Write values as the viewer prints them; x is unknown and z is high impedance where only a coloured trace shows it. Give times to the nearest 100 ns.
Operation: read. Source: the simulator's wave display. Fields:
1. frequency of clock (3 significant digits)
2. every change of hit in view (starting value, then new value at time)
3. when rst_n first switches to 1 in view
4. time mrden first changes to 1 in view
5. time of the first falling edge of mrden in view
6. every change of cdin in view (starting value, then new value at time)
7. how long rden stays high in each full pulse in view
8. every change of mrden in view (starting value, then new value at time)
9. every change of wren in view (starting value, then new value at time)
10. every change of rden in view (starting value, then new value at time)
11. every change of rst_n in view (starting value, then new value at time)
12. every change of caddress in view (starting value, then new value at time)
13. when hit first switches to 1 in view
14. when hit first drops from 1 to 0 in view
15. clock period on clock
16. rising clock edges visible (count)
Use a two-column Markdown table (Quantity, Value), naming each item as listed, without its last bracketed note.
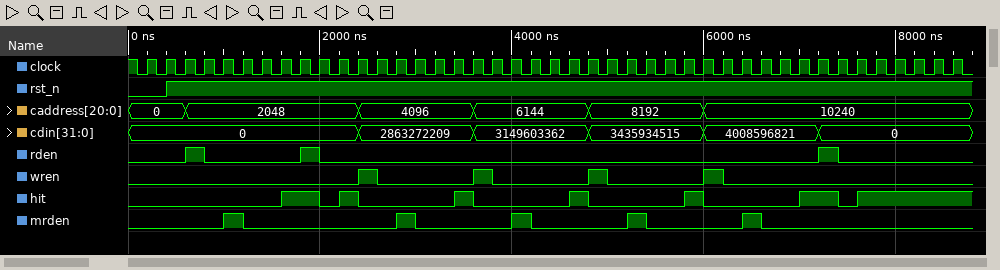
| Quantity | Value |
|---|---|
| frequency of clock | 5.00 MHz |
| every change of hit in view | 0, 1 at 1600 ns, 0 at 2000 ns, 1 at 2200 ns, 0 at 2400 ns, 1 at 3400 ns, 0 at 3600 ns, 1 at 4600 ns, 0 at 4800 ns, 1 at 5800 ns, 0 at 6000 ns, 1 at 7000 ns, 0 at 7400 ns, 1 at 7600 ns |
| when rst_n first switches to 1 in view | 400 ns |
| time mrden first changes to 1 in view | 1000 ns |
| time of the first falling edge of mrden in view | 1200 ns |
| every change of cdin in view | 0, 2863272209 at 2400 ns, 3149603362 at 3600 ns, 3435934515 at 4800 ns, 4008596821 at 6000 ns, 0 at 7200 ns |
| how long rden stays high in each full pulse in view | 200 ns, 200 ns, 200 ns |
| every change of mrden in view | 0, 1 at 1000 ns, 0 at 1200 ns, 1 at 2800 ns, 0 at 3000 ns, 1 at 4000 ns, 0 at 4200 ns, 1 at 5200 ns, 0 at 5400 ns, 1 at 6400 ns, 0 at 6600 ns |
| every change of wren in view | 0, 1 at 2400 ns, 0 at 2600 ns, 1 at 3600 ns, 0 at 3800 ns, 1 at 4800 ns, 0 at 5000 ns, 1 at 6000 ns, 0 at 6200 ns |
| every change of rden in view | 0, 1 at 600 ns, 0 at 800 ns, 1 at 1800 ns, 0 at 2000 ns, 1 at 7200 ns, 0 at 7400 ns |
| every change of rst_n in view | 0, 1 at 400 ns |
| every change of caddress in view | 0, 2048 at 600 ns, 4096 at 2400 ns, 6144 at 3600 ns, 8192 at 4800 ns, 10240 at 6000 ns |
| when hit first switches to 1 in view | 1600 ns |
| when hit first drops from 1 to 0 in view | 2000 ns |
| clock period on clock | 200 ns |
| rising clock edges visible | 43 |
